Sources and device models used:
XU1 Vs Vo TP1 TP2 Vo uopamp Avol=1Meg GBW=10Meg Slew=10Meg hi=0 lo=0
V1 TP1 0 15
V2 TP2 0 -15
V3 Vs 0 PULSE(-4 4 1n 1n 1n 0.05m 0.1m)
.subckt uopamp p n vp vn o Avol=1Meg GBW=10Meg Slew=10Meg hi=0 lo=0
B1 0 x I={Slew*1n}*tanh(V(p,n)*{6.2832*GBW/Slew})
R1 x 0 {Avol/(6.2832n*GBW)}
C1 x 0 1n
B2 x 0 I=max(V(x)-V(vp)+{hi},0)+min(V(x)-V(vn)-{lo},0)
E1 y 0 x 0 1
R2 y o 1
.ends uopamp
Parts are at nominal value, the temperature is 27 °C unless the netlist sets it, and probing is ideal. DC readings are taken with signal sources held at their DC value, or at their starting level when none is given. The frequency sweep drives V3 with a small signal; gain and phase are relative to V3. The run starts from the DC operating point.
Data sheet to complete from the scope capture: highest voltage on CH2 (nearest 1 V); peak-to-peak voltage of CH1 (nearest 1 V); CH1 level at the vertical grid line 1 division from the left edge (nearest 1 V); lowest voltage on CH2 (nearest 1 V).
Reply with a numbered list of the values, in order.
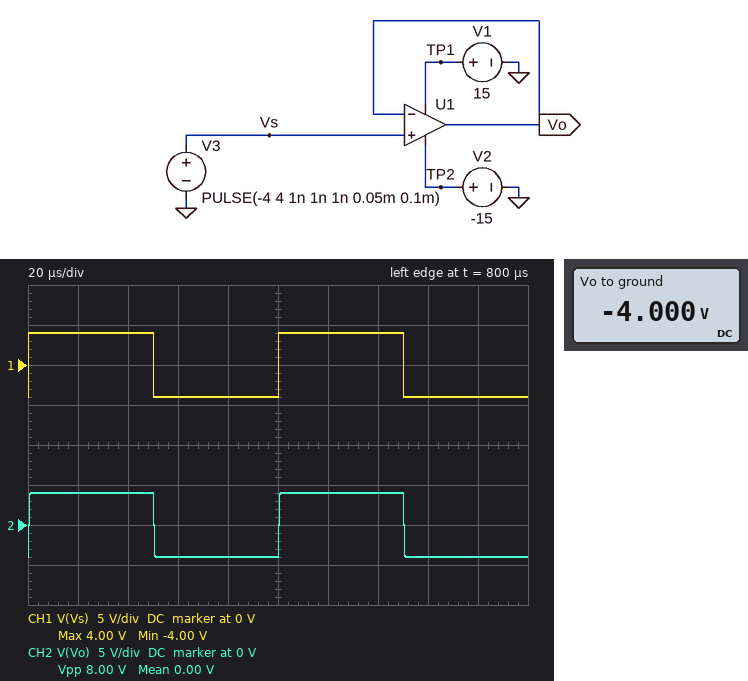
1. 4 V
2. 8 V
3. 4 V
4. -4 V
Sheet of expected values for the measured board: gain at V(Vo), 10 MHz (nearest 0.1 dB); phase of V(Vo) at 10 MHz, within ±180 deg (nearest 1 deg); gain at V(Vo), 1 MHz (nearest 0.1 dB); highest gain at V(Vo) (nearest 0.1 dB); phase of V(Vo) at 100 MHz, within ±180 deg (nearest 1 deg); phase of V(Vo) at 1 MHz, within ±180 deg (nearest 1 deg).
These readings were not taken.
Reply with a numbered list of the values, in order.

1. -3.0 dB
2. -45 deg
3. 0 dB
4. 0 dB
5. -84 deg
6. -6 deg
